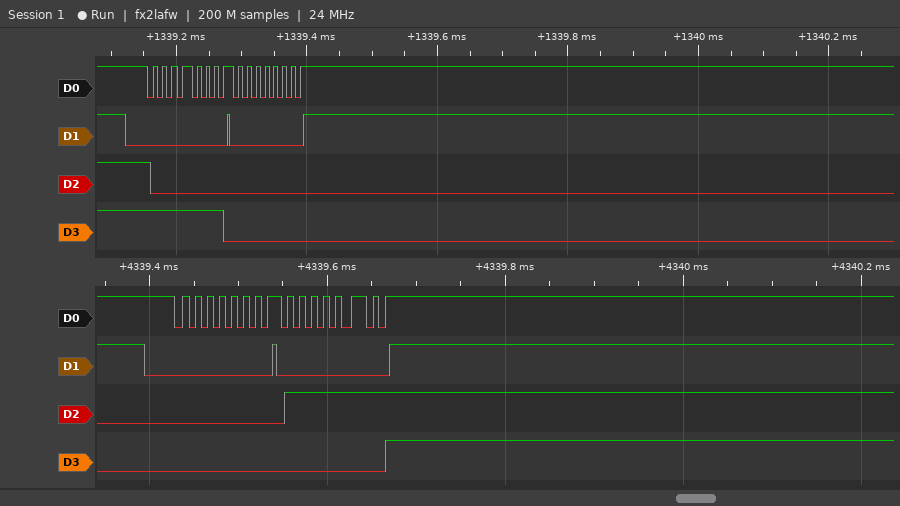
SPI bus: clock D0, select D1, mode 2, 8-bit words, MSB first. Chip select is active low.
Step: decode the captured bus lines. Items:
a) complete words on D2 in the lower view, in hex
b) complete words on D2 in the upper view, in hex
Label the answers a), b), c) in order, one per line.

a) 00, 7F
b) 80, 00
